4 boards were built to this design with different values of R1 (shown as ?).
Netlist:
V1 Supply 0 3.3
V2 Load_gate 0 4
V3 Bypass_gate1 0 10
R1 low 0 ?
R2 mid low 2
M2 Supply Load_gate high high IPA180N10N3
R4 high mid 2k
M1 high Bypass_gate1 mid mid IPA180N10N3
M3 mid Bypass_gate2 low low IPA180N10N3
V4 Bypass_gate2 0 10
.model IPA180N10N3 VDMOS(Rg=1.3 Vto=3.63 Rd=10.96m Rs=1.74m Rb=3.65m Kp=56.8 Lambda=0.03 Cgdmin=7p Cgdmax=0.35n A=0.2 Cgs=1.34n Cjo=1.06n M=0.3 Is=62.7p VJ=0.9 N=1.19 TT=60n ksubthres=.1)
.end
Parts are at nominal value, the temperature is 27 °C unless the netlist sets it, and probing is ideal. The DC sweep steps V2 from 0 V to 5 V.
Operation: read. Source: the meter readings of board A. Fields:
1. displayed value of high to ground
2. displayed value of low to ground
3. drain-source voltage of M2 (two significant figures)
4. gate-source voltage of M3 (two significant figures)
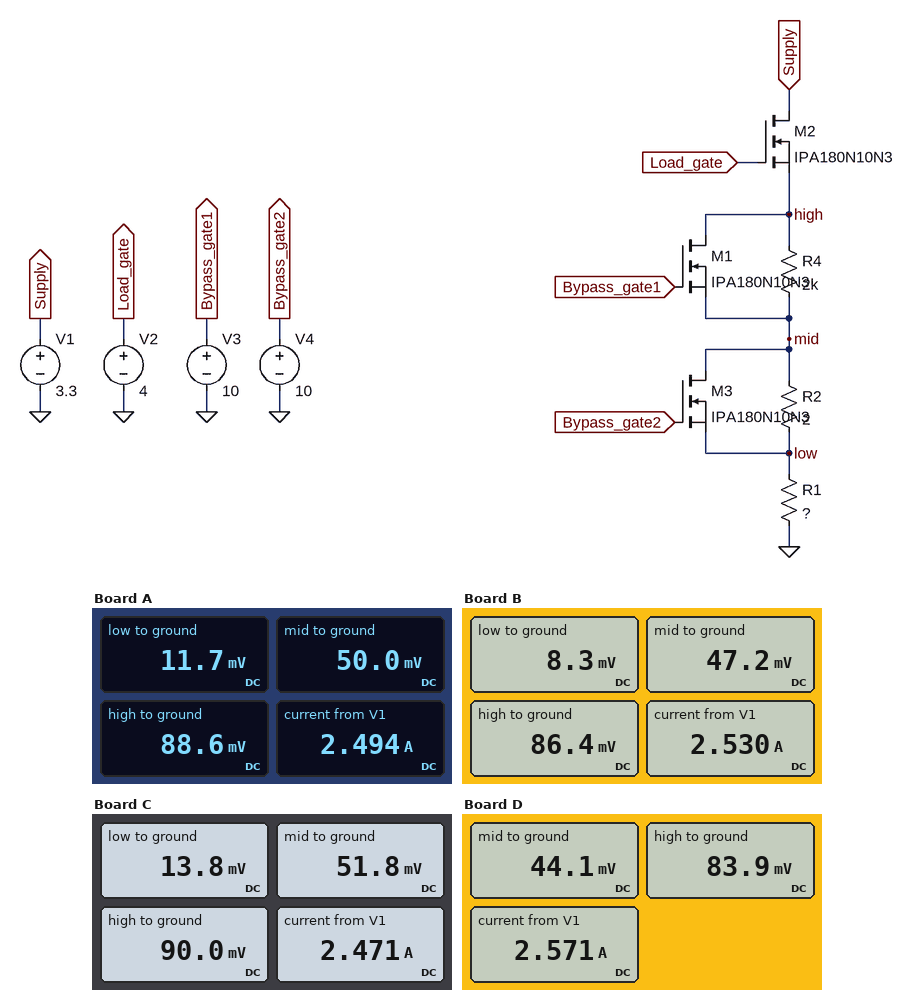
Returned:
88.6 mV
11.7 mV
3.2 V
10 V
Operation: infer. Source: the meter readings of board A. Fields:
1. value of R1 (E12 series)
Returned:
4.7 mΩ
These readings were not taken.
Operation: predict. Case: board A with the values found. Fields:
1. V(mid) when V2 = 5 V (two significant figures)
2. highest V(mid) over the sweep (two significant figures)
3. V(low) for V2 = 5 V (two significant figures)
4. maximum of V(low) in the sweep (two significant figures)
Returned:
340 mV
340 mV
79 mV
79 mV
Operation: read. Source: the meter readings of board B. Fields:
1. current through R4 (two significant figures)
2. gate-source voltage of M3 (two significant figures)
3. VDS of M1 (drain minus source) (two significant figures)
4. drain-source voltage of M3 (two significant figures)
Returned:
20 µA
10 V
39 mV
39 mV
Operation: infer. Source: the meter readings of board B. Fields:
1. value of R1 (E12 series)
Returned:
3.3 mΩ
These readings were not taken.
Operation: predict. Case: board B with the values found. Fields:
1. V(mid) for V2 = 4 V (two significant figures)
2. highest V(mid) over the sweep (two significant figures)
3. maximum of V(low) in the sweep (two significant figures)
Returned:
47 mV
320 mV
57 mV
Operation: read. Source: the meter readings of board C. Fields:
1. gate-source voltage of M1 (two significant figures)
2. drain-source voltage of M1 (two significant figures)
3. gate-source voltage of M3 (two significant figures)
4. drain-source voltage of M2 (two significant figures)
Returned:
9.9 V
38 mV
10 V
3.2 V
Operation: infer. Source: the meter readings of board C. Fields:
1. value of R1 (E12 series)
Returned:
5.6 mΩ
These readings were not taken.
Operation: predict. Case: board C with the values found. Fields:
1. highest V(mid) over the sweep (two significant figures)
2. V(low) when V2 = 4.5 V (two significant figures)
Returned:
350 mV
49 mV
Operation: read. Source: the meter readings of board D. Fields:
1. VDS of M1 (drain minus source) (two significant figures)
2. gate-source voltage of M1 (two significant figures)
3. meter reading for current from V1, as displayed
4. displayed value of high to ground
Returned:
40 mV
10 V
2.571 A
83.9 mV
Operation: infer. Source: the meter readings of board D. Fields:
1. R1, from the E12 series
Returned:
1.8 mΩ
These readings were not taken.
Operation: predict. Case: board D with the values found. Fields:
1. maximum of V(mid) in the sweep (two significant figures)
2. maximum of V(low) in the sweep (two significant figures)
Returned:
300 mV
32 mV
